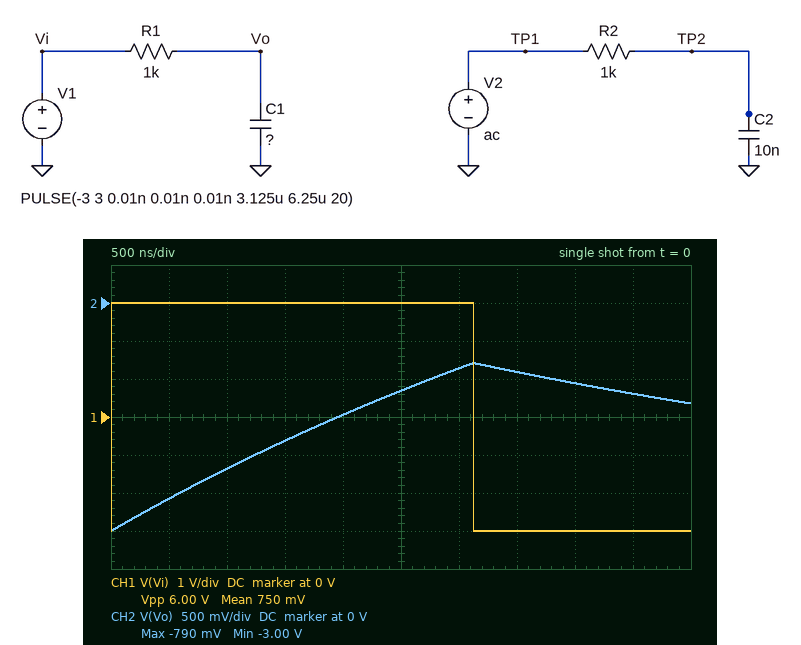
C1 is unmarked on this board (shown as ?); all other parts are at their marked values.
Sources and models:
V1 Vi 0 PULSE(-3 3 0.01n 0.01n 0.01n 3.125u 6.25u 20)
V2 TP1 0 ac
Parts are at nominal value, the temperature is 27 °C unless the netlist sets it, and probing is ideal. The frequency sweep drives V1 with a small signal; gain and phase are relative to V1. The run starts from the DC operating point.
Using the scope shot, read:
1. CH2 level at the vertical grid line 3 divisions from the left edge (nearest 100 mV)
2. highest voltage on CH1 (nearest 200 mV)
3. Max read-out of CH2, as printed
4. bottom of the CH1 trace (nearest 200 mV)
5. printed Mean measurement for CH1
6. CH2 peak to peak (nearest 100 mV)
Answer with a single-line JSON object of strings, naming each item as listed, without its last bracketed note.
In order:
{"CH2 level at the vertical grid line 3 divisions from the left edge": "-1.8 V", "highest voltage on CH1": "3.0 V", "Max read-out of CH2, as printed": "-790 mV", "bottom of the CH1 trace": "-3.0 V", "printed Mean measurement for CH1": "750 mV", "CH2 peak to peak": "2.2 V"}
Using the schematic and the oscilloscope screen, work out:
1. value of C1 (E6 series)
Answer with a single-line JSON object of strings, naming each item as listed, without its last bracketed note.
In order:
{"value of C1": "6.8 nF"}
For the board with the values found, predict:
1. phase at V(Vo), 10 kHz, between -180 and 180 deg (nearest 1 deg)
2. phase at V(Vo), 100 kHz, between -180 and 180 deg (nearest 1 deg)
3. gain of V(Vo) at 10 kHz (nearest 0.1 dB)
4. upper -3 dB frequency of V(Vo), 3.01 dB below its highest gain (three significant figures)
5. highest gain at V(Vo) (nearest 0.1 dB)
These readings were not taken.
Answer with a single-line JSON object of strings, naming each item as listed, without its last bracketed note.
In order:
{"phase at V(Vo), 10 kHz, between -180 and 180 deg": "-23 deg", "phase at V(Vo), 100 kHz, between -180 and 180 deg": "-77 deg", "gain of V(Vo) at 10 kHz": "-0.7 dB", "upper -3 dB frequency of V(Vo), 3.01 dB below its highest gain": "23.4 kHz", "highest gain at V(Vo)": "0 dB"}
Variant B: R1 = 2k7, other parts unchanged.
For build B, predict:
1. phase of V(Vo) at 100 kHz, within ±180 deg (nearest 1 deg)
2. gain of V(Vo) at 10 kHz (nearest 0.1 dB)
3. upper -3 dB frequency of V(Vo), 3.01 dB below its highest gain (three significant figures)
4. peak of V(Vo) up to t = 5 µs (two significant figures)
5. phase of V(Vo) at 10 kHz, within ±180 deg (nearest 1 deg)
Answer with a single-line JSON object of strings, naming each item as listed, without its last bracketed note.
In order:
{"phase of V(Vo) at 100 kHz, within ±180 deg": "-85 deg", "gain of V(Vo) at 10 kHz": "-3.7 dB", "upper -3 dB frequency of V(Vo), 3.01 dB below its highest gain": "8.67 kHz", "peak of V(Vo) up to t = 5 µs": "-2.1 V", "phase of V(Vo) at 10 kHz, within ±180 deg": "-49 deg"}
